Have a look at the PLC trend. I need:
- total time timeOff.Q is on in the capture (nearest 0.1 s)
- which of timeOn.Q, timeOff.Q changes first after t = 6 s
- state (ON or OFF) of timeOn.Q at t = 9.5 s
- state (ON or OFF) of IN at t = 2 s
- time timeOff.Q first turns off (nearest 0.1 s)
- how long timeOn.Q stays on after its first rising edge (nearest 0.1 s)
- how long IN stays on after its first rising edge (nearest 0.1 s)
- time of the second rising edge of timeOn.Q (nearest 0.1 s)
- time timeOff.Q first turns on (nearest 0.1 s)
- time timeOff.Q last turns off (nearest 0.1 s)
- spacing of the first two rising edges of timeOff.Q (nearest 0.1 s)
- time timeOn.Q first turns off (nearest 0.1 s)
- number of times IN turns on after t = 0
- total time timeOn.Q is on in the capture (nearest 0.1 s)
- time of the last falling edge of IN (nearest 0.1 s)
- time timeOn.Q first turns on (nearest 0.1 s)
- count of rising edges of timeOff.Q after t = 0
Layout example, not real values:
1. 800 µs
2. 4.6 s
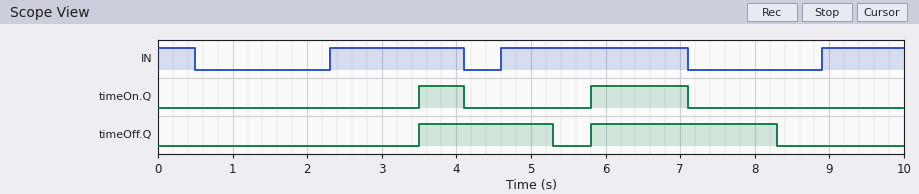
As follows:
1. 4.3 s
2. timeOn.Q
3. OFF
4. OFF
5. 5.3 s
6. 0.6 s
7. 1.8 s
8. 5.8 s
9. 3.5 s
10. 8.3 s
11. 2.3 s
12. 4.1 s
13. 3
14. 1.9 s
15. 7.1 s
16. 3.5 s
17. 2
